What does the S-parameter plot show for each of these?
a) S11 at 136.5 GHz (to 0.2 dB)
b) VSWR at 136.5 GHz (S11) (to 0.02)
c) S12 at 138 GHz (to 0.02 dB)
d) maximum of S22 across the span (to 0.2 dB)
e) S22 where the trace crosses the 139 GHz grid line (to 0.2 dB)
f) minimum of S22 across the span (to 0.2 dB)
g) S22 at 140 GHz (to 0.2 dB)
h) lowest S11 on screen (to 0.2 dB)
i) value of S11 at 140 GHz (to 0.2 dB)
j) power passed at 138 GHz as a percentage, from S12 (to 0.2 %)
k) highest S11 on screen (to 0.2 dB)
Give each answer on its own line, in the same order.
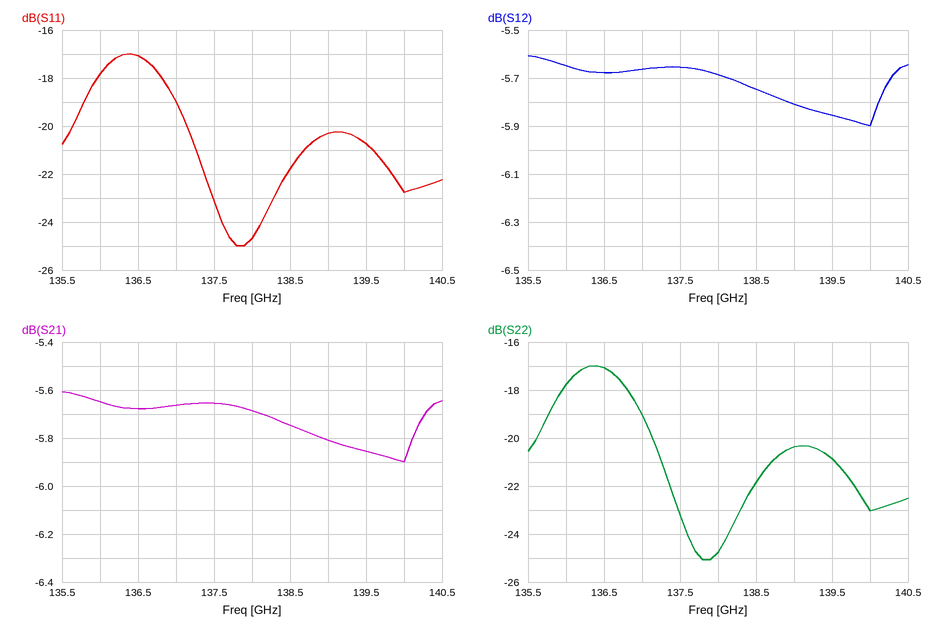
-17.0 dB
1.32
-5.68 dB
-17.0 dB
-20.4 dB
-25.0 dB
-23.0 dB
-25.0 dB
-22.8 dB
27.0 %
-17.0 dB
